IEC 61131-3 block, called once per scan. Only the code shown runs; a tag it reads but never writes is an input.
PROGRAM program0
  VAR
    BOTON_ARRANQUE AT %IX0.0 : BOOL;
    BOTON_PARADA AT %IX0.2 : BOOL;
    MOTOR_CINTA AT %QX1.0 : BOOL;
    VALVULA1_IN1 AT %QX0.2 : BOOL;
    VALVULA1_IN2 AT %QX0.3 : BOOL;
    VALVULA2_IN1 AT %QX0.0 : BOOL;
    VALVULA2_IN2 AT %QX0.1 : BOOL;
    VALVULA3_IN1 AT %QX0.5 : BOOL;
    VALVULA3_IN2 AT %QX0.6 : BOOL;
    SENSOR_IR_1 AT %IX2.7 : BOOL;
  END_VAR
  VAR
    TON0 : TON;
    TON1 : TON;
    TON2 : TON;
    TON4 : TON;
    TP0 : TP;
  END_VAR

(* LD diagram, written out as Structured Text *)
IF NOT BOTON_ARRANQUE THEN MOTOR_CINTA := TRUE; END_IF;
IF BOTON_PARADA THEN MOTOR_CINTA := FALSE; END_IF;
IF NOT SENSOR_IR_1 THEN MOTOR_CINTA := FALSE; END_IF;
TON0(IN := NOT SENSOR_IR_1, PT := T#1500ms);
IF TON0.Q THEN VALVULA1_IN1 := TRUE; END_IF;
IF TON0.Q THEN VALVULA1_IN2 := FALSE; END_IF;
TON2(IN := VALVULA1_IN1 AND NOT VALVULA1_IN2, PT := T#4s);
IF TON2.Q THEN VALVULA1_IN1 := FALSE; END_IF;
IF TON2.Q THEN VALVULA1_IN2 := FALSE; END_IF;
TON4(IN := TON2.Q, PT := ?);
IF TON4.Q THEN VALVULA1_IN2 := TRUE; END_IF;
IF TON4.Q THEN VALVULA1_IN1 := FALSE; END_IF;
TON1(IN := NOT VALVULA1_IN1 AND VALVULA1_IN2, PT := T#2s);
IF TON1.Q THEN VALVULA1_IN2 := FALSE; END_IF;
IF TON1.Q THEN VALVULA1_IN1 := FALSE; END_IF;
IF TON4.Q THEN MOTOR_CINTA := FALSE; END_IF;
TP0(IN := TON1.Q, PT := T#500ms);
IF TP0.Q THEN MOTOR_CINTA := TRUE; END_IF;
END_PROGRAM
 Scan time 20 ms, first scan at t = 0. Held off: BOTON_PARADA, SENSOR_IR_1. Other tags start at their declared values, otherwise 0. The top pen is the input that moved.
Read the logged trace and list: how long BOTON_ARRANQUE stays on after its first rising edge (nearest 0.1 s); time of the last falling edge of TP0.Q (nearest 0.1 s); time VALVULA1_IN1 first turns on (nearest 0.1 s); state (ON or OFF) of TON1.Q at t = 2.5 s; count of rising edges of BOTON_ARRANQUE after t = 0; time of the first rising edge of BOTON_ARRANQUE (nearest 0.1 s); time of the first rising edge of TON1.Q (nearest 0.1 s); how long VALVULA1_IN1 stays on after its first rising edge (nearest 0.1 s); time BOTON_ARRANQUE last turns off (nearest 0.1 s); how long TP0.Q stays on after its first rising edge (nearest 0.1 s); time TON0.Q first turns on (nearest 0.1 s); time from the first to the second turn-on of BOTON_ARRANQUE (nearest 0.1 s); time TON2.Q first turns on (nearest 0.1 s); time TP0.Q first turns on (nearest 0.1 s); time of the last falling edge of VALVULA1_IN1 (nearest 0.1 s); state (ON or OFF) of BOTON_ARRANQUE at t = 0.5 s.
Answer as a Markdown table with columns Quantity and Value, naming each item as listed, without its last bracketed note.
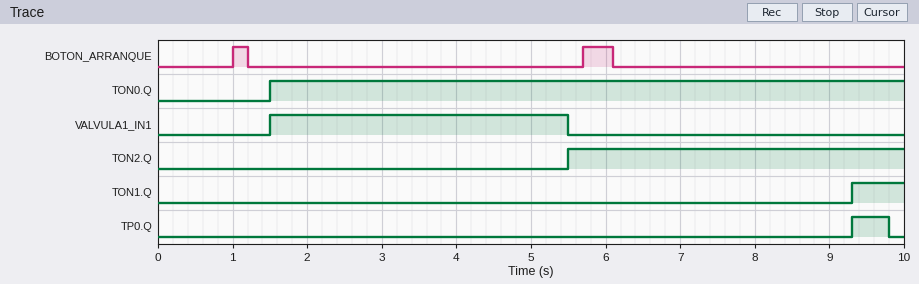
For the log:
| Quantity | Value |
|---|---|
| how long BOTON_ARRANQUE stays on after its first rising edge | 0.2 s |
| time of the last falling edge of TP0.Q | 9.8 s |
| time VALVULA1_IN1 first turns on | 1.5 s |
| state (ON or OFF) of TON1.Q at t = 2.5 s | OFF |
| count of rising edges of BOTON_ARRANQUE after t = 0 | 2 |
| time of the first rising edge of BOTON_ARRANQUE | 1.0 s |
| time of the first rising edge of TON1.Q | 9.3 s |
| how long VALVULA1_IN1 stays on after its first rising edge | 4.0 s |
| time BOTON_ARRANQUE last turns off | 6.1 s |
| how long TP0.Q stays on after its first rising edge | 0.5 s |
| time TON0.Q first turns on | 1.5 s |
| time from the first to the second turn-on of BOTON_ARRANQUE | 4.7 s |
| time TON2.Q first turns on | 5.5 s |
| time TP0.Q first turns on | 9.3 s |
| time of the last falling edge of VALVULA1_IN1 | 5.5 s |
| state (ON or OFF) of BOTON_ARRANQUE at t = 0.5 s | OFF |
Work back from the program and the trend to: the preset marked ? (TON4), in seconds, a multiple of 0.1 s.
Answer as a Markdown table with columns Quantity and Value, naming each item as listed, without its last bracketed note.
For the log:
| Quantity | Value |
|---|---|
| the preset marked ? (TON4), in seconds, a multiple of 0.1 s | 1.8 s |
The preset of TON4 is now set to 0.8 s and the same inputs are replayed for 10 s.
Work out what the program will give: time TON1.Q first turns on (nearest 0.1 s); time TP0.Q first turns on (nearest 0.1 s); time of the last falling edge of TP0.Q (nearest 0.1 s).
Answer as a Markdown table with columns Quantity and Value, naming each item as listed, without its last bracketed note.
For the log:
| Quantity | Value |
|---|---|
| time TON1.Q first turns on | 8.3 s |
| time TP0.Q first turns on | 8.3 s |
| time of the last falling edge of TP0.Q | 8.8 s |
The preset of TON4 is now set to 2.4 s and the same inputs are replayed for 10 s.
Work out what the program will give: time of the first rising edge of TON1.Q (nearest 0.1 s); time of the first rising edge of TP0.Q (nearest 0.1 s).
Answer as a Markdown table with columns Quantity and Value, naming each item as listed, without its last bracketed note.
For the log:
| Quantity | Value |
|---|---|
| time of the first rising edge of TON1.Q | 9.9 s |
| time of the first rising edge of TP0.Q | 9.9 s |
